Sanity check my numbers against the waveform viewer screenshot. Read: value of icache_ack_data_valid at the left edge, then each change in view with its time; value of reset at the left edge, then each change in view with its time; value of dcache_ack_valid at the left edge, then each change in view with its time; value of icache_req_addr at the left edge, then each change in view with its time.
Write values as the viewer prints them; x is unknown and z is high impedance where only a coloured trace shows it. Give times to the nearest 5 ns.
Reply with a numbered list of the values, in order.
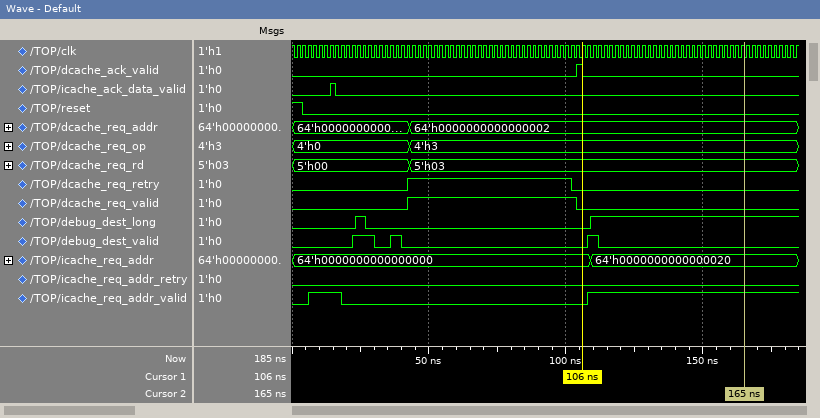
1. 0, 1 at 15 ns, 0 at 15 ns
2. 1, 0 at 5 ns
3. 0, 1 at 105 ns, 0 at 105 ns
4. 64'h0000000000000000, 64'h0000000000000020 at 110 ns
